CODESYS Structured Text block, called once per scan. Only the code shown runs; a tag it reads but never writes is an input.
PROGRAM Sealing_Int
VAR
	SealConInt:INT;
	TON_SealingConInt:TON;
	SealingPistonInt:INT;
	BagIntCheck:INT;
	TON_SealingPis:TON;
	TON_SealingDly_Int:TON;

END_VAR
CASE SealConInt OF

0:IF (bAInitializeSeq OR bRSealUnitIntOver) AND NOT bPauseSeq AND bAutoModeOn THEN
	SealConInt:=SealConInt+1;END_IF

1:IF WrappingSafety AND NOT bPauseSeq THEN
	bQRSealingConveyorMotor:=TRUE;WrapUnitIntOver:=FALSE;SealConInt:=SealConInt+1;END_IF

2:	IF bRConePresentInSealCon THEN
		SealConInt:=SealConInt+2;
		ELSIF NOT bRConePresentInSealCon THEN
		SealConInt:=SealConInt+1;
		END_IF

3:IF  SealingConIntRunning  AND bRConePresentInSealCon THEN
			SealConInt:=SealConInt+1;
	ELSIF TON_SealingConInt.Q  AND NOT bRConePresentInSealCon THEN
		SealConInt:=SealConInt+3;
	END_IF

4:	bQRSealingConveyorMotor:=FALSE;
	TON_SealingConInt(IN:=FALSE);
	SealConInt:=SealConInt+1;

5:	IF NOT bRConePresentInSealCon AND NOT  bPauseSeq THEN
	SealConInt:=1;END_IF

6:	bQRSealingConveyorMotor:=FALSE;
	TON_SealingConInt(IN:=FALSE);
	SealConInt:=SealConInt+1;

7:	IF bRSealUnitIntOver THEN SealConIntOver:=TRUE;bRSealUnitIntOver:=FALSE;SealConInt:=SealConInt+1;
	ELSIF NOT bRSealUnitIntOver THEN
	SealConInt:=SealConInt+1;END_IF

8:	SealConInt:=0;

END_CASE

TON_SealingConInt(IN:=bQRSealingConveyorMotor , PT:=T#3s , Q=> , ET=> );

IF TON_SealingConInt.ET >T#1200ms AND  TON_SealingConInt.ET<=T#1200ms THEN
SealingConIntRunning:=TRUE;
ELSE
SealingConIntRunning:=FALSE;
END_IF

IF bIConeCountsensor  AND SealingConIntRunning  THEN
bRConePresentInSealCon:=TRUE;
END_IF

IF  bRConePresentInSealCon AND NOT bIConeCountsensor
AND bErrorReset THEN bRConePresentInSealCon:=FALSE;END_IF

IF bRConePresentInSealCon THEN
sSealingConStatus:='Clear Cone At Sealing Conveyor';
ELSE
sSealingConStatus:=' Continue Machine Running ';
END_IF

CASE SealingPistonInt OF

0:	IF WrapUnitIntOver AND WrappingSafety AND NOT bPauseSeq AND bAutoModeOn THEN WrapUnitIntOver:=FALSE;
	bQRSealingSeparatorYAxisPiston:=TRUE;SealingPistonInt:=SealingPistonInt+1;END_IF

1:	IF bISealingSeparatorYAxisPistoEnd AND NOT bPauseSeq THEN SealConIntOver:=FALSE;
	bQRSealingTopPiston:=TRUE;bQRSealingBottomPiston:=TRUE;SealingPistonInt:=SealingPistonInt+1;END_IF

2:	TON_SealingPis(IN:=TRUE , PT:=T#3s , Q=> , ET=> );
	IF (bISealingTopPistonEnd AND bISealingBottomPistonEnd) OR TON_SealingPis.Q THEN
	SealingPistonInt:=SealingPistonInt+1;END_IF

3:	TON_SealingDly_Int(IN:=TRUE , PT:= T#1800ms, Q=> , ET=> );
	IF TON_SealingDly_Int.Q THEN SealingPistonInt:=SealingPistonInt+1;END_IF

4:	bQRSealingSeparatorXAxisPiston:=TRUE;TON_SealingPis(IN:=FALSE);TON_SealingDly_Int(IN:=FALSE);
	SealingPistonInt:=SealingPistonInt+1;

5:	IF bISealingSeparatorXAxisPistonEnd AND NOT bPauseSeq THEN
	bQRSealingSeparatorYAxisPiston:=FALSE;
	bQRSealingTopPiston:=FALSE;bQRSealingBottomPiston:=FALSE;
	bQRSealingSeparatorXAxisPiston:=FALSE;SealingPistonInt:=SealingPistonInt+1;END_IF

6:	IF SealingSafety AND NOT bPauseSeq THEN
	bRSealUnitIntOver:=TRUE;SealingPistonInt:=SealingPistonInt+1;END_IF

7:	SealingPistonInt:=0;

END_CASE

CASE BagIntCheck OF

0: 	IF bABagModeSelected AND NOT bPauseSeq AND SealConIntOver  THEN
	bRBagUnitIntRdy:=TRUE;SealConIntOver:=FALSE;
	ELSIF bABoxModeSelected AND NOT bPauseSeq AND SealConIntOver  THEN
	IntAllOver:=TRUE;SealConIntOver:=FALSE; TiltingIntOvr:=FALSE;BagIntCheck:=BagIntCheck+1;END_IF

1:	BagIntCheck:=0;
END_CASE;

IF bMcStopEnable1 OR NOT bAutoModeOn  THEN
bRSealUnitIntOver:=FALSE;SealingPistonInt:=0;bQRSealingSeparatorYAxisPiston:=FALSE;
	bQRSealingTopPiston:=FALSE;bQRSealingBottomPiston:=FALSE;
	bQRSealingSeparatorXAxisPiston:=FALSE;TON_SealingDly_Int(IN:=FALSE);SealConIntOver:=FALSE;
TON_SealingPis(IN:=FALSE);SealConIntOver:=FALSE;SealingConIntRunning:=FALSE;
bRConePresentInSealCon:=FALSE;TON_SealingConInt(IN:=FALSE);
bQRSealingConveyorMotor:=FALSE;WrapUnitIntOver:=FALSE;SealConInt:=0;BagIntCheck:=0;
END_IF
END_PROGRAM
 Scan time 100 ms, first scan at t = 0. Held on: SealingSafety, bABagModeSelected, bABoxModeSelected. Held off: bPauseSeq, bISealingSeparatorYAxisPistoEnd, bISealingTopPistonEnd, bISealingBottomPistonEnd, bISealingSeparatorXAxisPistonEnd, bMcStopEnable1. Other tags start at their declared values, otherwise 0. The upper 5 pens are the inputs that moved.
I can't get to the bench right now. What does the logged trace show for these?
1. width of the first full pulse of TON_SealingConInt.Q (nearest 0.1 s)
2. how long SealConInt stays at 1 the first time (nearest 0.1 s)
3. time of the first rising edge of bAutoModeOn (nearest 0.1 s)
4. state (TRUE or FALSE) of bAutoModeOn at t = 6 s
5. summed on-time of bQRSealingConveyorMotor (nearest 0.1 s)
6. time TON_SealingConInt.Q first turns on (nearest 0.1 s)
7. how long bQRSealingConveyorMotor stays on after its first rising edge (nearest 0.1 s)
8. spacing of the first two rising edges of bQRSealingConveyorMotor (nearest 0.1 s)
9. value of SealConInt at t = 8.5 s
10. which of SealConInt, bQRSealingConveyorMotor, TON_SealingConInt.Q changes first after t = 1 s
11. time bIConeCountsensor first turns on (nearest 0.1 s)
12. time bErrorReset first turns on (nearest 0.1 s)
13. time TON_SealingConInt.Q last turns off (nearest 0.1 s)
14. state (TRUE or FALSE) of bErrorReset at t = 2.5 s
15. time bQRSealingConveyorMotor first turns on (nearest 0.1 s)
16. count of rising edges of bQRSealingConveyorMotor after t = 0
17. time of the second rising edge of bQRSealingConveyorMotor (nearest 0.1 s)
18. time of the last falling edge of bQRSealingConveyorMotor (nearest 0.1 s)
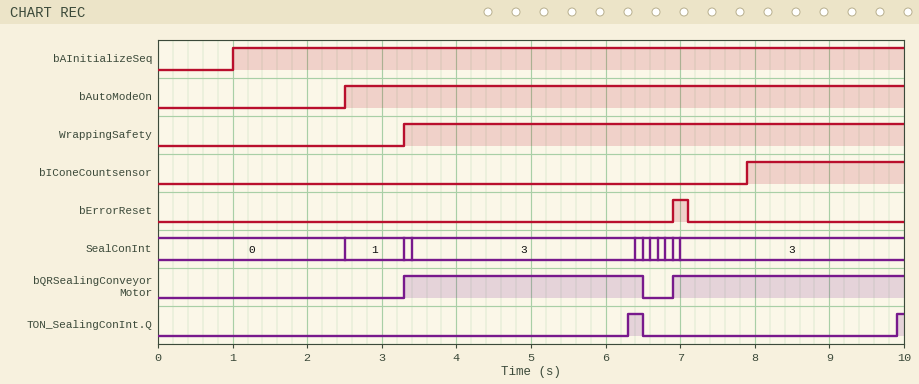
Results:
0.2 s
0.8 s
2.5 s
TRUE
6.3 s
6.3 s
3.2 s
3.6 s
3
SealConInt
7.9 s
6.9 s
6.5 s
FALSE
3.3 s
2
6.9 s
6.5 s
